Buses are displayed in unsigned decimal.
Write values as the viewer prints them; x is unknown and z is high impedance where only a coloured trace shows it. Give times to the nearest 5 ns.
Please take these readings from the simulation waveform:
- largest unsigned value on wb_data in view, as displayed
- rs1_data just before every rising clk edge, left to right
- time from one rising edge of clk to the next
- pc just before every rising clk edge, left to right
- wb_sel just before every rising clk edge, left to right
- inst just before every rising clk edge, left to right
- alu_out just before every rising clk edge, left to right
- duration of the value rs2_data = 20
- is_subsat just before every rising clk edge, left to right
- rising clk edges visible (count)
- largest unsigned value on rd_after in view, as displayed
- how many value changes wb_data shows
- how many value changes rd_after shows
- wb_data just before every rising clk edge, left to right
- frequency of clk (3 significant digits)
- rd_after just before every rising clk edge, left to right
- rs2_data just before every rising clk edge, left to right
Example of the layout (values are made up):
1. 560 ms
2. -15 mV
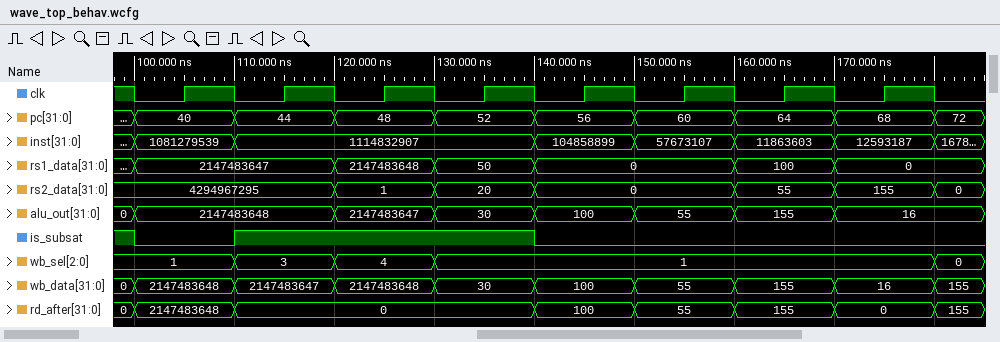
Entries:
1. 2147483648
2. 2147483647, 2147483647, 2147483648, 50, 0, 0, 100, 0
3. 10 ns
4. 40, 44, 48, 52, 56, 60, 64, 68
5. 1, 3, 4, 1, 1, 1, 1, 1
6. 1081279539, 1114832907, 1114832907, 1114832907, 104858899, 57673107, 11863603, 12593187
7. 2147483648, 2147483648, 2147483647, 30, 100, 55, 155, 16
8. 10 ns
9. 0 1 1 1 0 0 0 0
10. 8
11. 2147483648
12. 9
13. 7
14. 2147483648, 2147483647, 2147483648, 30, 100, 55, 155, 16
15. 100 MHz
16. 2147483648, 0, 0, 0, 100, 55, 155, 0
17. 4294967295, 4294967295, 1, 20, 0, 0, 55, 155
